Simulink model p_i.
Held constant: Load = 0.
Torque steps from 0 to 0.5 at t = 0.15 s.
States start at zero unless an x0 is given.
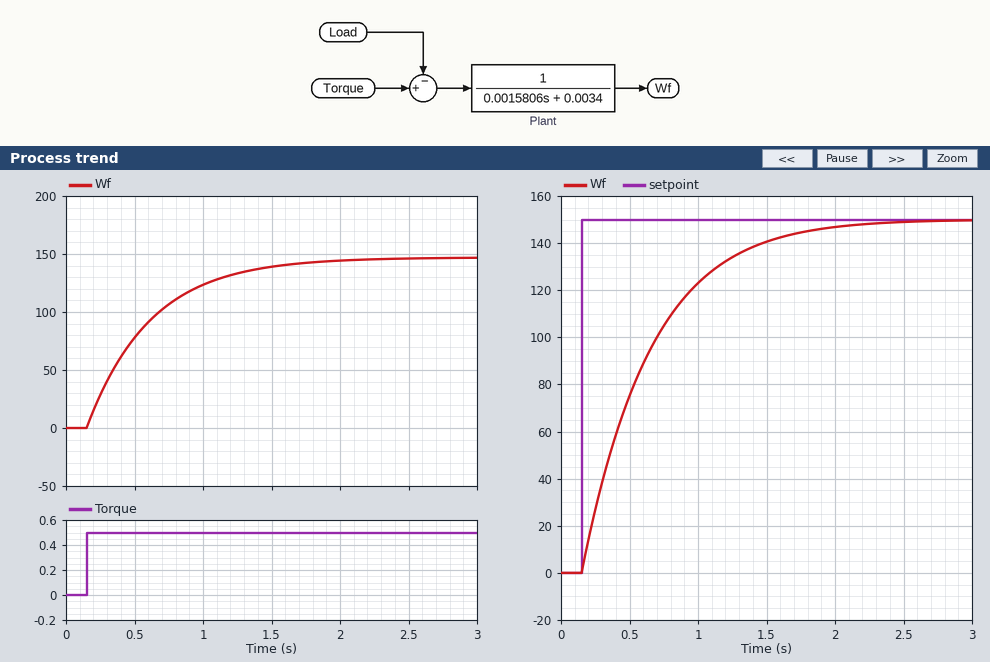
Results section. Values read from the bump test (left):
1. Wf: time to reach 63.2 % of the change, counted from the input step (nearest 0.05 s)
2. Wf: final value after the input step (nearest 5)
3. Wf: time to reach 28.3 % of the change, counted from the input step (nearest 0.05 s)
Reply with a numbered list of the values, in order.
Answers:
1. 0.45 s
2. 145
3. 0.15 s
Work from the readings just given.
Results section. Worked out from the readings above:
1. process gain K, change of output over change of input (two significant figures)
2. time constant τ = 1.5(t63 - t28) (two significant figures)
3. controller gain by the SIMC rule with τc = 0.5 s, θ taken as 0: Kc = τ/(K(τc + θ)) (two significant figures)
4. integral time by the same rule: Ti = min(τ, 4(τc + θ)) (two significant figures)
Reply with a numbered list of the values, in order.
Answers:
1. 290
2. 0.45 s
3. 0.0031
4. 0.45 s
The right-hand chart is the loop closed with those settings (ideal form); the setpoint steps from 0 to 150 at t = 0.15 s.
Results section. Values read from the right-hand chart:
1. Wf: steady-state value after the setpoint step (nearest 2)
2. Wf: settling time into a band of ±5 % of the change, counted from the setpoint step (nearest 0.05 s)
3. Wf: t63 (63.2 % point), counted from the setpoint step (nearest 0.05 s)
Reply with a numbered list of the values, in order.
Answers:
1. 150
2. 1.45 s
3. 0.50 s
